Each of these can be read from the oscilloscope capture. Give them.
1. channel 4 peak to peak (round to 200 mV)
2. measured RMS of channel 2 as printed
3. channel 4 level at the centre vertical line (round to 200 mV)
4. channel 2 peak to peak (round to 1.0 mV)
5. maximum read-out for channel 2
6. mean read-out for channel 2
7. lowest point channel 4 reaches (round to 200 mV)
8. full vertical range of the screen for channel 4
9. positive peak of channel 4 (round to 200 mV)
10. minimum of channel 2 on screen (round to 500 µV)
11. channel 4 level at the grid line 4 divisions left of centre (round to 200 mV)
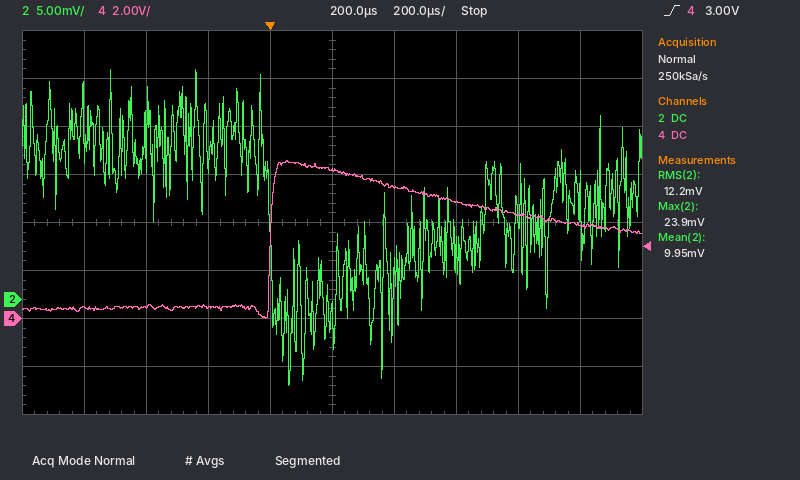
6.6 V
12.2 mV
6.2 V
33.0 mV
23.9 mV
9.95 mV
0.0 V
16 V
6.6 V
-9.0 mV
400 mV
